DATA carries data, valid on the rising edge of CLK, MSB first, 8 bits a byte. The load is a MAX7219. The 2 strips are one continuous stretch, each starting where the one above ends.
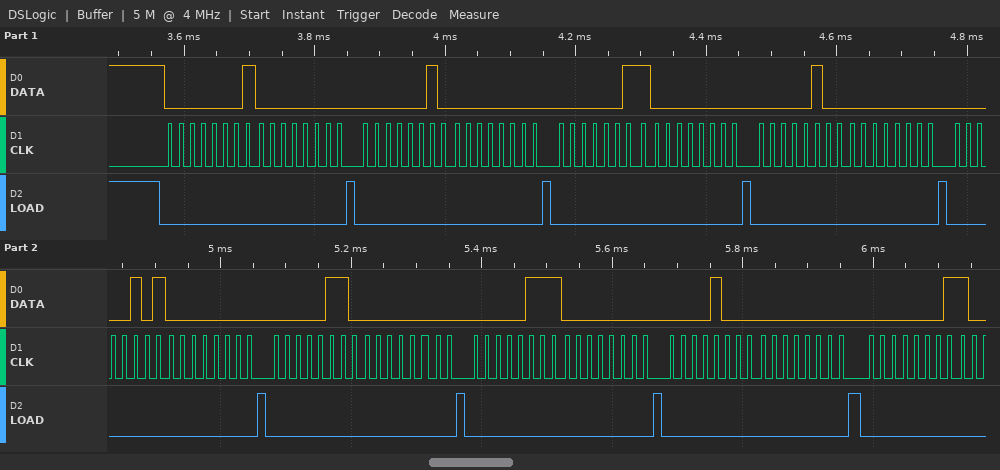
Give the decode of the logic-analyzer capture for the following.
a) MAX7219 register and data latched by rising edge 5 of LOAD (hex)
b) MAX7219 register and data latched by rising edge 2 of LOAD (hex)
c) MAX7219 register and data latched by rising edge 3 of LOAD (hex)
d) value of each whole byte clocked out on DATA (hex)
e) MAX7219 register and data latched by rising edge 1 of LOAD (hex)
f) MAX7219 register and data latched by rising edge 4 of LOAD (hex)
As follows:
register 0x5, data 0x00
register 0x2, data 0x00
register 0x3, data 0x00
01 00 02 00 03 00 04 00 05 00 06 00 07 00 08 00 01
register 0x1, data 0x00
register 0x4, data 0x00
